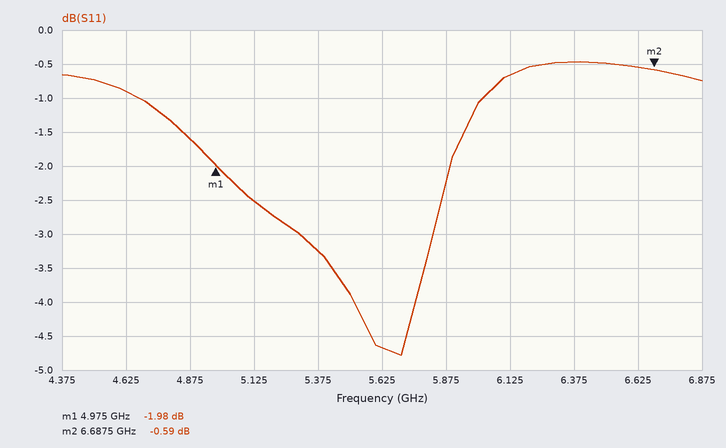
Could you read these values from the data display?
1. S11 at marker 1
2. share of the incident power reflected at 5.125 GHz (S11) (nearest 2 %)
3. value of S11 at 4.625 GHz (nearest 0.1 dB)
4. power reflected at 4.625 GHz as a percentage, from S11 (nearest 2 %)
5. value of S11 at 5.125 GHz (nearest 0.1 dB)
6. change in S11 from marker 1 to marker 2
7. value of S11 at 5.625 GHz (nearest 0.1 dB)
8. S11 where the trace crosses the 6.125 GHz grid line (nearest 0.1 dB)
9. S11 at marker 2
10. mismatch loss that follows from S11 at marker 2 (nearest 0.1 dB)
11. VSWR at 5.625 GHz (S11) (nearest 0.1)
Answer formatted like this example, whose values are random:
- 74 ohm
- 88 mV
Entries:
- -1.98 dB
- 56 %
- -0.9 dB
- 82 %
- -2.5 dB
- 1.39 dB
- -4.7 dB
- -0.7 dB
- -0.59 dB
- 9.0 dB
- 3.8
